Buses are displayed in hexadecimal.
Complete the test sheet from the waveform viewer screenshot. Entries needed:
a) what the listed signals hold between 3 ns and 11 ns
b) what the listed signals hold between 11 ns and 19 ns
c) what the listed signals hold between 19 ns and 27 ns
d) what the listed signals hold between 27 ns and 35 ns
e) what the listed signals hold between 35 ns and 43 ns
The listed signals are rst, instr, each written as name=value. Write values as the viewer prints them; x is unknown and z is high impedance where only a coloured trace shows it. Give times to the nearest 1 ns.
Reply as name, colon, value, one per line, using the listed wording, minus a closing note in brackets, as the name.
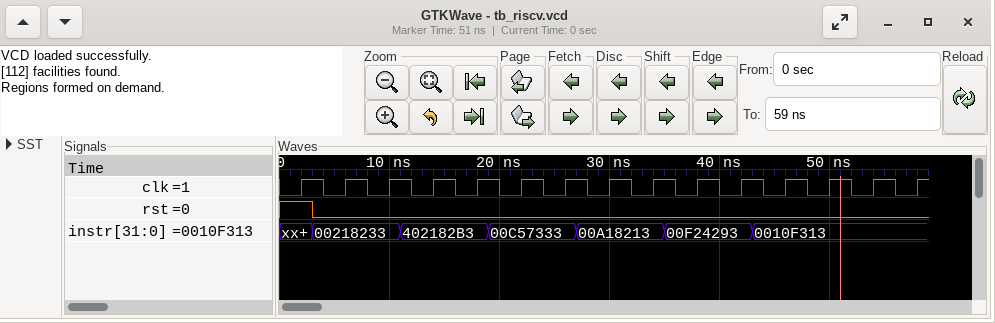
what the listed signals hold between 3 ns and 11 ns: rst=0, instr=00218233
what the listed signals hold between 11 ns and 19 ns: rst=0, instr=402182B3
what the listed signals hold between 19 ns and 27 ns: rst=0, instr=00C57333
what the listed signals hold between 27 ns and 35 ns: rst=0, instr=00A18213
what the listed signals hold between 35 ns and 43 ns: rst=0, instr=00F24293
